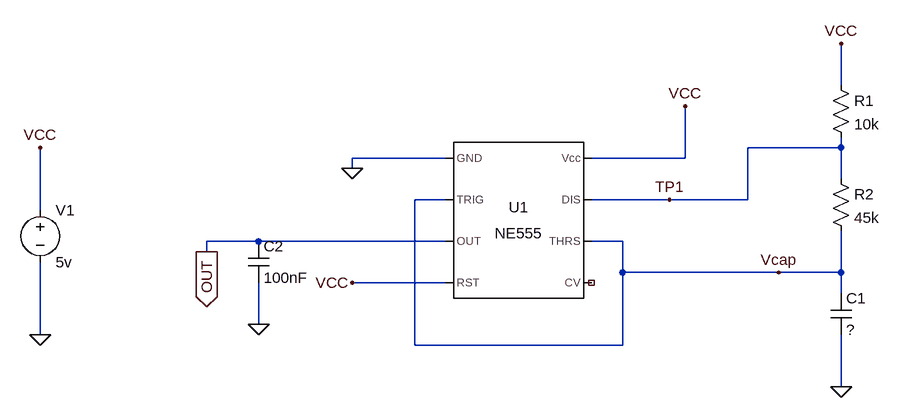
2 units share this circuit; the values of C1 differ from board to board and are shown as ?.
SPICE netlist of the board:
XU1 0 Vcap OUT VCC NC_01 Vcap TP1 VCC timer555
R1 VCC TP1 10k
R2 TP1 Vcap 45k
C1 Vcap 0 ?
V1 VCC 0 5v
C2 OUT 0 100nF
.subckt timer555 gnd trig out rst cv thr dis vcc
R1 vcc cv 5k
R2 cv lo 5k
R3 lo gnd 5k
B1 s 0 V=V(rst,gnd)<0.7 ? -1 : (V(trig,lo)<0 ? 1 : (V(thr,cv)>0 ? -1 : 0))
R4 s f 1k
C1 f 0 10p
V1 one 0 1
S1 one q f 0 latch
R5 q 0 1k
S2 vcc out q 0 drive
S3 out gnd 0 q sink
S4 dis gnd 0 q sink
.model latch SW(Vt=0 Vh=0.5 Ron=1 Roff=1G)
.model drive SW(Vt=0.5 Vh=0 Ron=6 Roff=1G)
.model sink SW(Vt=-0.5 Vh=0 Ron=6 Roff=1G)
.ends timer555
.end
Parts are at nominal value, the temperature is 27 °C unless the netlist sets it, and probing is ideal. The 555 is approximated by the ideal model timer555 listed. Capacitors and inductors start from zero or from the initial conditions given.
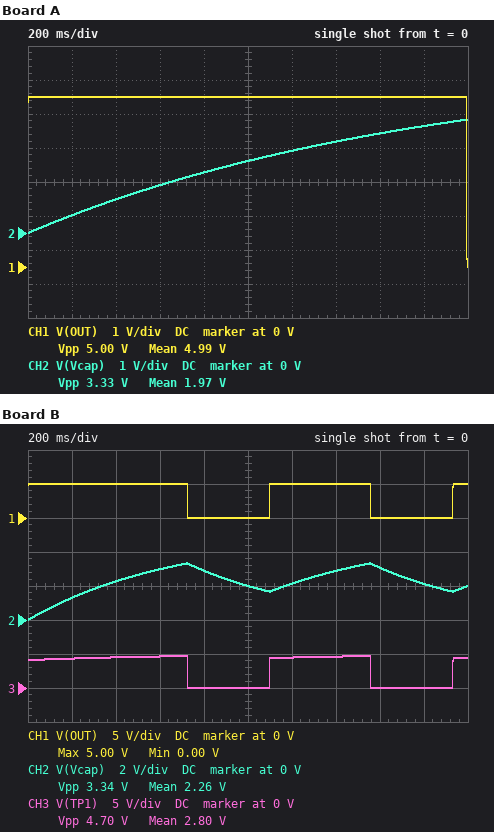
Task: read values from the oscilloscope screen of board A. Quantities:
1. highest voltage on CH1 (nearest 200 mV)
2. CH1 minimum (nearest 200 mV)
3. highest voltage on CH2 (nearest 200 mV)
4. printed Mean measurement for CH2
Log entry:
5.0 V
0 V
3.4 V
1.97 V
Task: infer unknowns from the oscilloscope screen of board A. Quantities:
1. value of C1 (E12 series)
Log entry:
33 µF
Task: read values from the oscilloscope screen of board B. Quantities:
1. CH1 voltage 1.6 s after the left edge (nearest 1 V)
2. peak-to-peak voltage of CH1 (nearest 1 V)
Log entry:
0 V
5 V
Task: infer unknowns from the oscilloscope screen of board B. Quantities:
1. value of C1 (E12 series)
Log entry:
12 µF
